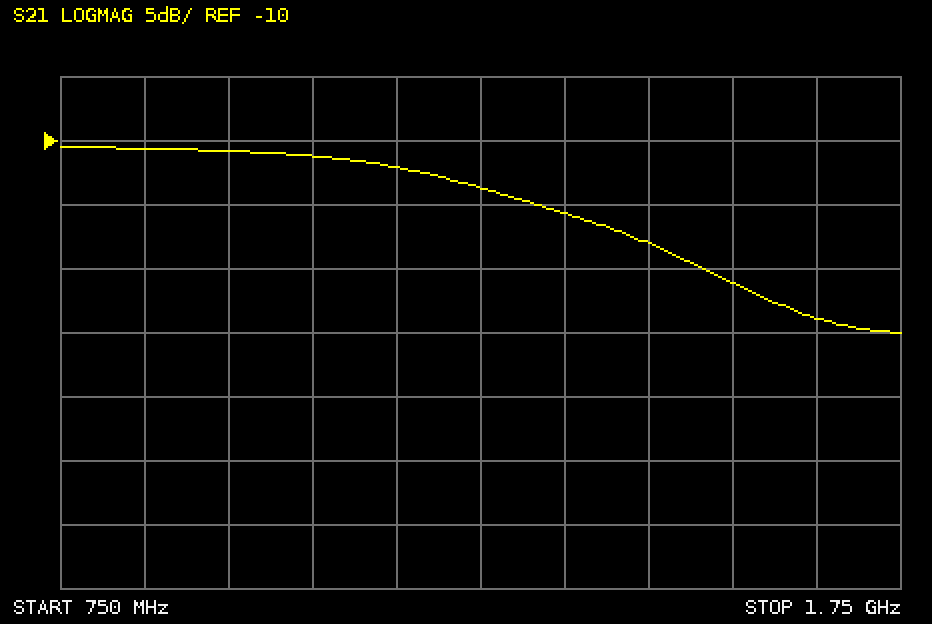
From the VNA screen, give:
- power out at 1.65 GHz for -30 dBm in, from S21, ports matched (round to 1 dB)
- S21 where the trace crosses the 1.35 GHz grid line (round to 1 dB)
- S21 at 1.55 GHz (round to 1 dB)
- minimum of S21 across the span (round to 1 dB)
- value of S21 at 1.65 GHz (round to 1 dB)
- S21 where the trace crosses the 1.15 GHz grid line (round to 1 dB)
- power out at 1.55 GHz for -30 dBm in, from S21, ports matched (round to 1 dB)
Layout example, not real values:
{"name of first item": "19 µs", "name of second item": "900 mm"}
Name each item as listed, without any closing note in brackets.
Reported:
{"power out at 1.65 GHz for -30 dBm in, from S21, ports matched": "-54 dBm", "S21 where the trace crosses the 1.35 GHz grid line": "-16 dB", "S21 at 1.55 GHz": "-21 dB", "minimum of S21 across the span": "-25 dB", "value of S21 at 1.65 GHz": "-24 dB", "S21 where the trace crosses the 1.15 GHz grid line": "-12 dB", "power out at 1.55 GHz for -30 dBm in, from S21, ports matched": "-51 dBm"}
